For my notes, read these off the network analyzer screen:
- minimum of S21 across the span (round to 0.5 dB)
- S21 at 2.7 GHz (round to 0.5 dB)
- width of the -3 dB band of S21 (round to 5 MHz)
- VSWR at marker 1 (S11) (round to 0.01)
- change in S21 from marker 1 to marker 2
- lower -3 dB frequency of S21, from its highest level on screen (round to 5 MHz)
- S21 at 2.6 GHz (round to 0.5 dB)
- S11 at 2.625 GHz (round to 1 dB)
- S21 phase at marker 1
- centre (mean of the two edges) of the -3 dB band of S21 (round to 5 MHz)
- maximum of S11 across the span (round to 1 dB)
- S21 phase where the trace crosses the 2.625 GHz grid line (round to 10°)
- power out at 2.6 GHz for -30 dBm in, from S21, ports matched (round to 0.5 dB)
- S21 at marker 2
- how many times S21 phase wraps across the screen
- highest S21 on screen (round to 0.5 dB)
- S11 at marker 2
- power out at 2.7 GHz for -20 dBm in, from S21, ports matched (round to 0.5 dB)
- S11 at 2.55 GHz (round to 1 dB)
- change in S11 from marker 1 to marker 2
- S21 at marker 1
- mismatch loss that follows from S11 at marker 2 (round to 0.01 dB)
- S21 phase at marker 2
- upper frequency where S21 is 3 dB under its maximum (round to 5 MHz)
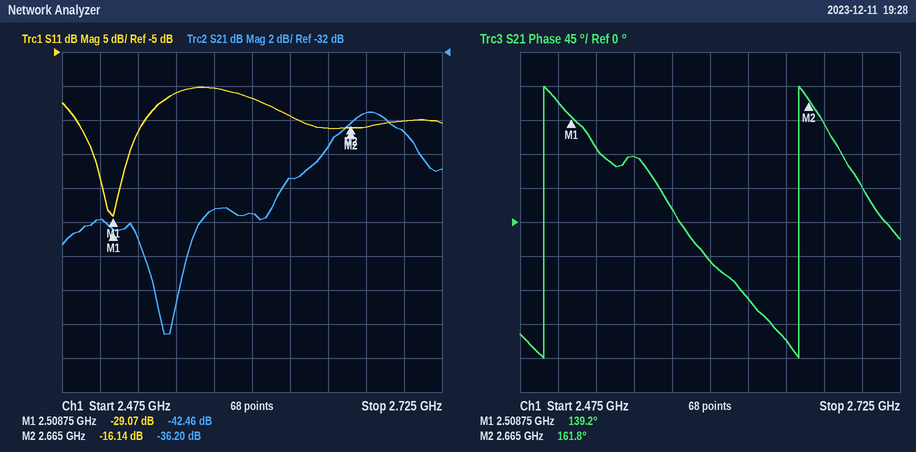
-48.5 dB
-36.5 dB
75 MHz
1.07
6.26 dB
2.640 GHz
-41.5 dB
-14 dB
139.2°
2.680 GHz
-10 dB
-100°
-71.5 dBm
-36.20 dB
2
-35.5 dB
-16.14 dB
-56.5 dBm
-11 dB
12.93 dB
-42.46 dB
0.11 dB
161.8°
2.715 GHz
